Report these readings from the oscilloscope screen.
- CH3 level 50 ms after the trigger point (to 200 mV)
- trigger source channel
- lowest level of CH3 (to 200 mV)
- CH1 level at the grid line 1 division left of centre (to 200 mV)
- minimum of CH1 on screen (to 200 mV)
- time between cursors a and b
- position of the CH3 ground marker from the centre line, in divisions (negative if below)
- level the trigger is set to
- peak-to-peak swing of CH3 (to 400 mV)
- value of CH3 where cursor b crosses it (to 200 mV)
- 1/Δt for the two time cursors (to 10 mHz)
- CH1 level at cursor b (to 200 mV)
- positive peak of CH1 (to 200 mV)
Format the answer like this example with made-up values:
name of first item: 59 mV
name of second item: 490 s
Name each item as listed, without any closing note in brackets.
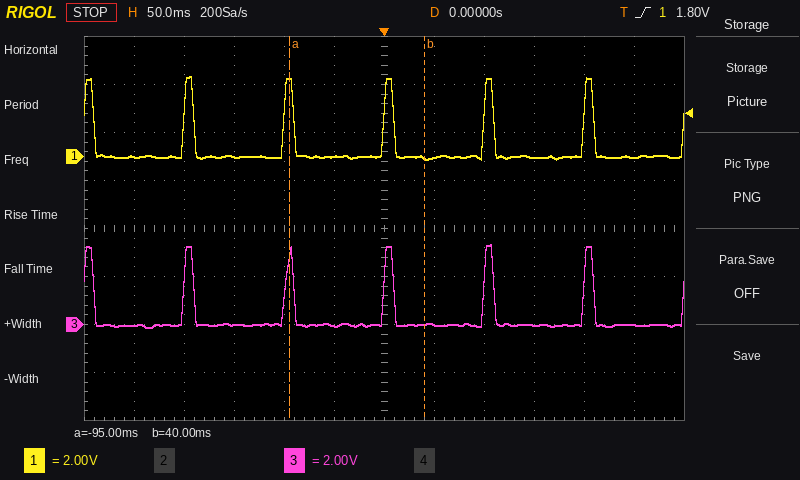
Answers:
CH3 level 50 ms after the trigger point: 0.0 V
trigger source channel: CH1
lowest level of CH3: -200 mV
CH1 level at the grid line 1 division left of centre: 0.0 V
minimum of CH1 on screen: -200 mV
time between cursors a and b: 135 ms
position of the CH3 ground marker from the centre line, in divisions: -2.0 div
level the trigger is set to: 1.80 V
peak-to-peak swing of CH3: 3.6 V
value of CH3 where cursor b crosses it: 0.0 V
1/Δt for the two time cursors: 7.41 Hz
CH1 level at cursor b: 0.0 V
positive peak of CH1: 3.4 V
